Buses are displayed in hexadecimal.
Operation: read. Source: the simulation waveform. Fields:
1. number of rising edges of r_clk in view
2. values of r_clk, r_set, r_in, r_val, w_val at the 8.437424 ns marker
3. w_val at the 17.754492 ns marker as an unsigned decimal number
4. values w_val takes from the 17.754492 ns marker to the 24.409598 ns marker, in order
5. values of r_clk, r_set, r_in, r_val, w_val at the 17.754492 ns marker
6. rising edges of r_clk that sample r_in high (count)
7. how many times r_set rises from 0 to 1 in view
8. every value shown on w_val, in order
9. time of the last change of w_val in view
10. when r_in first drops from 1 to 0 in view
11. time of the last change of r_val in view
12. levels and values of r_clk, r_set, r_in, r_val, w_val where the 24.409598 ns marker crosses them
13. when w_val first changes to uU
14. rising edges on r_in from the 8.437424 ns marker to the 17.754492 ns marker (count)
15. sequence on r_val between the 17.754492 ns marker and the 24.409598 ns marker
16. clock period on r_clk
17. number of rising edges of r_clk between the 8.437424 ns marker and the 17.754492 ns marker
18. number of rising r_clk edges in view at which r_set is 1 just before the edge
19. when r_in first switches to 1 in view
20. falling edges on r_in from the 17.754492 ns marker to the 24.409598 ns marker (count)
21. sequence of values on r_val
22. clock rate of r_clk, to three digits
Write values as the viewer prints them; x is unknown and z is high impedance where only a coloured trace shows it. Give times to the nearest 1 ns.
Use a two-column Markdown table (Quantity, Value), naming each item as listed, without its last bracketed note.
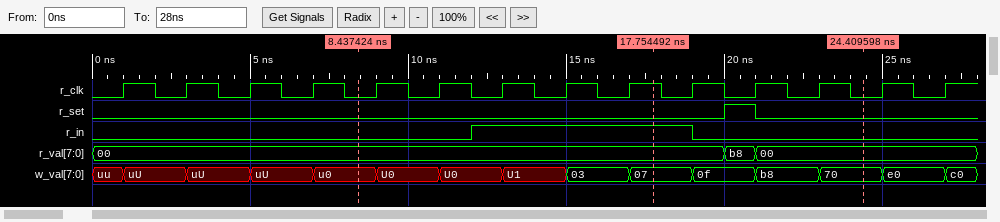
| Quantity | Value |
|---|---|
| number of rising edges of r_clk in view | 14 |
| values of r_clk, r_set, r_in, r_val, w_val at the 8.437424 ns marker | r_clk=0, r_set=0, r_in=0, r_val=00, w_val=u0 |
| w_val at the 17.754492 ns marker as an unsigned decimal number | 7 |
| values w_val takes from the 17.754492 ns marker to the 24.409598 ns marker, in order | 07, 0f, b8, 70 |
| values of r_clk, r_set, r_in, r_val, w_val at the 17.754492 ns marker | r_clk=1, r_set=0, r_in=1, r_val=00, w_val=07 |
| rising edges of r_clk that sample r_in high | 4 |
| how many times r_set rises from 0 to 1 in view | 1 |
| every value shown on w_val, in order | uu, uU, uU, uU, u0, U0, U0, U1, 03, 07, 0f, b8, 70, e0, c0 |
| time of the last change of w_val in view | 27 ns |
| when r_in first drops from 1 to 0 in view | 19 ns |
| time of the last change of r_val in view | 21 ns |
| levels and values of r_clk, r_set, r_in, r_val, w_val where the 24.409598 ns marker crosses them | r_clk=0, r_set=0, r_in=0, r_val=00, w_val=70 |
| when w_val first changes to uU | 1 ns |
| rising edges on r_in from the 8.437424 ns marker to the 17.754492 ns marker | 1 |
| sequence on r_val between the 17.754492 ns marker and the 24.409598 ns marker | 00, b8, 00 |
| clock period on r_clk | 2 ns |
| number of rising edges of r_clk between the 8.437424 ns marker and the 17.754492 ns marker | 5 |
| number of rising r_clk edges in view at which r_set is 1 just before the edge | 1 |
| when r_in first switches to 1 in view | 12 ns |
| falling edges on r_in from the 17.754492 ns marker to the 24.409598 ns marker | 1 |
| sequence of values on r_val | 00, b8, 00 |
| clock rate of r_clk, to three digits | 500 MHz |
